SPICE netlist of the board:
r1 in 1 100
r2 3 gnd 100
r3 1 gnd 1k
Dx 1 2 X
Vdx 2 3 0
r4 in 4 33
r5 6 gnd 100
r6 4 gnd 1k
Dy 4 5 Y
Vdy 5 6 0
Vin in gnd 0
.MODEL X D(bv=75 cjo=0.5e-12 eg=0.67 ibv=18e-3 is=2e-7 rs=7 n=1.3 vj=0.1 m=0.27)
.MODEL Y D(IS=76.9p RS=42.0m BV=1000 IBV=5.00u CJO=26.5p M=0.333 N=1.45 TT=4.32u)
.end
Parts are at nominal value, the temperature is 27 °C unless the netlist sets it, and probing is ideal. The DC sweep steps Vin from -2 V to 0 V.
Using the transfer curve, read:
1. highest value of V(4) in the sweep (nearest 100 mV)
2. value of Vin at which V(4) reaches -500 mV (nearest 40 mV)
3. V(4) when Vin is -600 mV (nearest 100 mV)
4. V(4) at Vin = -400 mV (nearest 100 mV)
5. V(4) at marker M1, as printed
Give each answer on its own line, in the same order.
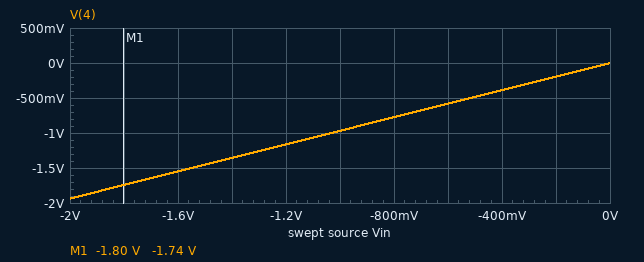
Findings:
0 V
-520 mV
-600 mV
-400 mV
-1.74 V
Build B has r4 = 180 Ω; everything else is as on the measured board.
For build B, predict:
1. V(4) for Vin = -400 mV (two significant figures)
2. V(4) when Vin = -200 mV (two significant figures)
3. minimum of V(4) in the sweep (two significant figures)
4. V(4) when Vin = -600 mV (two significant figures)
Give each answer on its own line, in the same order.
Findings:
-340 mV
-170 mV
-1.7 V
-510 mV
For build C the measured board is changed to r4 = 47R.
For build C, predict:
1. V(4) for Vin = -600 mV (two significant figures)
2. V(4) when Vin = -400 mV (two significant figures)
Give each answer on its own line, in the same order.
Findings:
-570 mV
-380 mV
